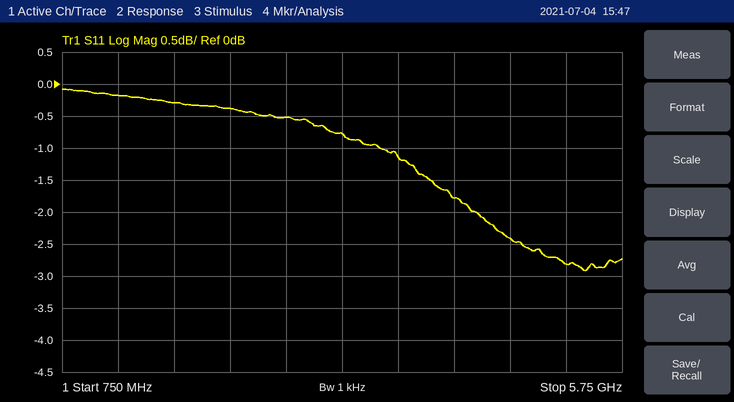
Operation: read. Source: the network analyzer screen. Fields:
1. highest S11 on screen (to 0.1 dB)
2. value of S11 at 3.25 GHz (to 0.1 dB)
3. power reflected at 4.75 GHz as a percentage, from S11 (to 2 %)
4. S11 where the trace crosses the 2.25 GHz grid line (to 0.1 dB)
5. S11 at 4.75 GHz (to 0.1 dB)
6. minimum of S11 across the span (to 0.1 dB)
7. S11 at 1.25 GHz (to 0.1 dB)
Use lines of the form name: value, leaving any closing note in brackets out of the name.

highest S11 on screen: -0.1 dB
value of S11 at 3.25 GHz: -0.8 dB
power reflected at 4.75 GHz as a percentage, from S11: 58 %
S11 where the trace crosses the 2.25 GHz grid line: -0.4 dB
S11 at 4.75 GHz: -2.4 dB
minimum of S11 across the span: -2.9 dB
S11 at 1.25 GHz: -0.2 dB
